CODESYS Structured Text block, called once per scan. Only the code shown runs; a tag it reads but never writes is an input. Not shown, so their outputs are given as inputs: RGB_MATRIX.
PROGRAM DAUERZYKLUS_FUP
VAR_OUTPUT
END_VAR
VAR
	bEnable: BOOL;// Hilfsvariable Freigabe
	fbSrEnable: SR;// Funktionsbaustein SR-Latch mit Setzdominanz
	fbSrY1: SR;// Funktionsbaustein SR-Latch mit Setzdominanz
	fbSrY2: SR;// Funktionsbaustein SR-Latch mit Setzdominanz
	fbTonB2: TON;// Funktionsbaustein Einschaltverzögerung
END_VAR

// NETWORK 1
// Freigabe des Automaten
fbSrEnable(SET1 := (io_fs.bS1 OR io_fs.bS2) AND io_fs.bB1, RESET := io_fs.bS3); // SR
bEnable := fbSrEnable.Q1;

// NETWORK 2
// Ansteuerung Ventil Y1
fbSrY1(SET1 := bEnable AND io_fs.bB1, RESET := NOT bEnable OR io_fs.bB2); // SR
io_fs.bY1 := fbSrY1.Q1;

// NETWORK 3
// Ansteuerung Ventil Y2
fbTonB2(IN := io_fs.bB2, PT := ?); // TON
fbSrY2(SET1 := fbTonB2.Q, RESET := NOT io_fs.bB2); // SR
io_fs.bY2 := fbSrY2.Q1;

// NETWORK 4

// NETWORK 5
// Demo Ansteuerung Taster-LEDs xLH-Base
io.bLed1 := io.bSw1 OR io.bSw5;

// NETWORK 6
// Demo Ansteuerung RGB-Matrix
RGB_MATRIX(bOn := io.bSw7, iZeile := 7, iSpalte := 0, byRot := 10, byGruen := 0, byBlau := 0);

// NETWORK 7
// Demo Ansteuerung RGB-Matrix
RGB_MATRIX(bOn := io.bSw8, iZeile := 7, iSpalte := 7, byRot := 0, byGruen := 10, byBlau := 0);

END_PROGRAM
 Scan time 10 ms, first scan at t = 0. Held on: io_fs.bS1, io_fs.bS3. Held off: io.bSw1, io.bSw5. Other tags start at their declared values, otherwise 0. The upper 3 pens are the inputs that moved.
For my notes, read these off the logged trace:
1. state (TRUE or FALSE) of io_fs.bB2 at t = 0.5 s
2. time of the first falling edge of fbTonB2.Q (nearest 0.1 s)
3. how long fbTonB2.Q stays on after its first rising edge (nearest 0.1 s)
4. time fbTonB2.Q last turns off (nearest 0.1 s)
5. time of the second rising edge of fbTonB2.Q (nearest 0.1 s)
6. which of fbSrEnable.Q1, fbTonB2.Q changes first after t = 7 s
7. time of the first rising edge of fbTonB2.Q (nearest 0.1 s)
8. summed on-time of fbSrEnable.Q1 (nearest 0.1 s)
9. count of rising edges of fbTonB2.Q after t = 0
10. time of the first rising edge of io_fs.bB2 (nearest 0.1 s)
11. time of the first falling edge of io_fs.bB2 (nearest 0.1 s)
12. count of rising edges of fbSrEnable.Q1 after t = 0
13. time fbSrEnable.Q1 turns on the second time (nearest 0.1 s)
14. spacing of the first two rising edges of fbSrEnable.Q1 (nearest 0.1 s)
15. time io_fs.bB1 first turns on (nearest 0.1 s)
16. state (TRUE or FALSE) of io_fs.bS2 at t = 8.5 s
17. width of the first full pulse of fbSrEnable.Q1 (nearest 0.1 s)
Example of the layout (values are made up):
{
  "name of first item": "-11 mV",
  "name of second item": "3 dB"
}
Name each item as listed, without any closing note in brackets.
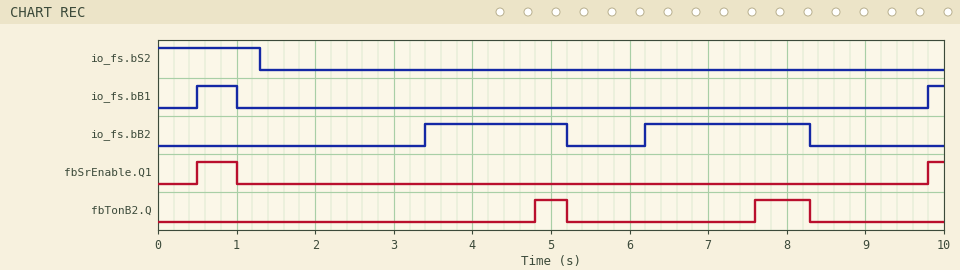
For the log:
{
  "state (TRUE or FALSE) of io_fs.bB2 at t = 0.5 s": "FALSE",
  "time of the first falling edge of fbTonB2.Q": "5.2 s",
  "how long fbTonB2.Q stays on after its first rising edge": "0.4 s",
  "time fbTonB2.Q last turns off": "8.3 s",
  "time of the second rising edge of fbTonB2.Q": "7.6 s",
  "which of fbSrEnable.Q1, fbTonB2.Q changes first after t = 7 s": "fbTonB2.Q",
  "time of the first rising edge of fbTonB2.Q": "4.8 s",
  "summed on-time of fbSrEnable.Q1": "0.7 s",
  "count of rising edges of fbTonB2.Q after t = 0": "2",
  "time of the first rising edge of io_fs.bB2": "3.4 s",
  "time of the first falling edge of io_fs.bB2": "5.2 s",
  "count of rising edges of fbSrEnable.Q1 after t = 0": "2",
  "time fbSrEnable.Q1 turns on the second time": "9.8 s",
  "spacing of the first two rising edges of fbSrEnable.Q1": "9.3 s",
  "time io_fs.bB1 first turns on": "0.5 s",
  "state (TRUE or FALSE) of io_fs.bS2 at t = 8.5 s": "FALSE",
  "width of the first full pulse of fbSrEnable.Q1": "0.5 s"
}
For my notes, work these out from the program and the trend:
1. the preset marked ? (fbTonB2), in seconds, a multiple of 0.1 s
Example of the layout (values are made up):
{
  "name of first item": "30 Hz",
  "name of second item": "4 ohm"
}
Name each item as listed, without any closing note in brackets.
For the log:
{
  "the preset marked ? (fbTonB2), in seconds, a multiple of 0.1 s": "1.4 s"
}
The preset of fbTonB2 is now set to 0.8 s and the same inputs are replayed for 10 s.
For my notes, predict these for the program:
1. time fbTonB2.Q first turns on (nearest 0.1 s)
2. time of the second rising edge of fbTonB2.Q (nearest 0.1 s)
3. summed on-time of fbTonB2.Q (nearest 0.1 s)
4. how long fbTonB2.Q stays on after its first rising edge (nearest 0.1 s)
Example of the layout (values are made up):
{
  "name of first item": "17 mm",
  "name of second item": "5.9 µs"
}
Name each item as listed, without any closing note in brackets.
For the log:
{
  "time fbTonB2.Q first turns on": "4.2 s",
  "time of the second rising edge of fbTonB2.Q": "7.0 s",
  "summed on-time of fbTonB2.Q": "2.3 s",
  "how long fbTonB2.Q stays on after its first rising edge": "1.0 s"
}
